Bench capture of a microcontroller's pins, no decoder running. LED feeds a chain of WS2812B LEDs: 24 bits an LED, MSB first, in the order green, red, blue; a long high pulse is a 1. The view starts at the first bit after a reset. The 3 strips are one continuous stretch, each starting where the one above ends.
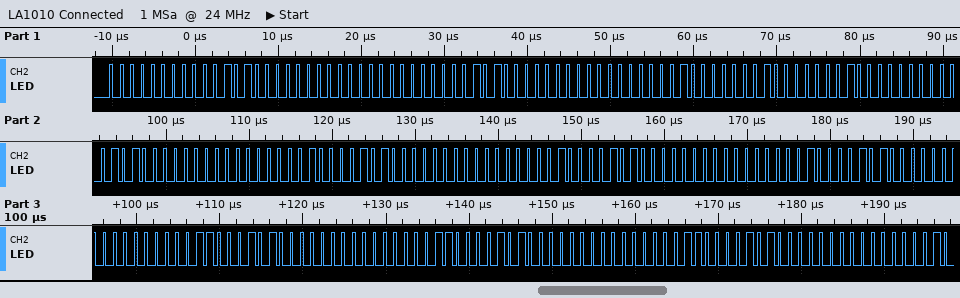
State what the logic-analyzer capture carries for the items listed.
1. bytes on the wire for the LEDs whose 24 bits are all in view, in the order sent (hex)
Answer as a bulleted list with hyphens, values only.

- 00 14 00 00 14 00 01 01 01 00 14 00 02 14 00 02 14 00 02 14 00 03 14 00 06 14 00 06 14 00
